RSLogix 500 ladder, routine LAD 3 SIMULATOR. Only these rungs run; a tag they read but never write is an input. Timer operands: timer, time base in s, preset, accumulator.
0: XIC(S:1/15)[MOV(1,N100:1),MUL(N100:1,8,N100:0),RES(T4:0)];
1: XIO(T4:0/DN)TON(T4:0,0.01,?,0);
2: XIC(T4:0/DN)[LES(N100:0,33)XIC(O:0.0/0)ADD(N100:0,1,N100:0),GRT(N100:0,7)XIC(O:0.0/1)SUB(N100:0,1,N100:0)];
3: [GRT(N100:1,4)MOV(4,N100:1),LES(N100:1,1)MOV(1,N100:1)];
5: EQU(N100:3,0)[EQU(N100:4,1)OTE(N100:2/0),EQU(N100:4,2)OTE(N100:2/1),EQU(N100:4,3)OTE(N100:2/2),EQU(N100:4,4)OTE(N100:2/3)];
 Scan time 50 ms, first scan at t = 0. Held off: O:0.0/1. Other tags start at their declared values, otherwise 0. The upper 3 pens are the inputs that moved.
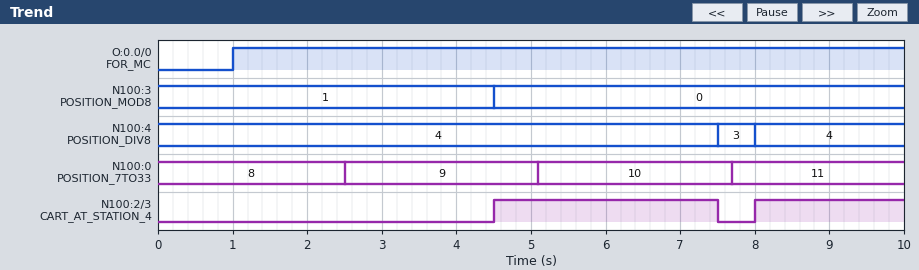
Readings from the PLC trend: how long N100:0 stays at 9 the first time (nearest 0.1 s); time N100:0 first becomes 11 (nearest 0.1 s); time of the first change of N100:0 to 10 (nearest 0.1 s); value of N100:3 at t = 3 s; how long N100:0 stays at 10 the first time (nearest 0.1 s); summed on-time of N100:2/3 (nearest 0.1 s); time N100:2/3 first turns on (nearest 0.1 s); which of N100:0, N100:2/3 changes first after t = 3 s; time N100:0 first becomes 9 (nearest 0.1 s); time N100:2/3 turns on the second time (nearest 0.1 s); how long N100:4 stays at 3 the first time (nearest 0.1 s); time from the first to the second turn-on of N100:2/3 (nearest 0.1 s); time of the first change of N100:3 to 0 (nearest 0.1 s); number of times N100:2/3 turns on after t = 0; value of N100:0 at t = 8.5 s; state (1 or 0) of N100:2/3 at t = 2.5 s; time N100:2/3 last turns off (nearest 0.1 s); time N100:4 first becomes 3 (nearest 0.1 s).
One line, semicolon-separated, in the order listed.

2.6 s; 7.7 s; 5.1 s; 1; 2.6 s; 5.0 s; 4.5 s; N100:2/3; 2.5 s; 8.0 s; 0.5 s; 3.5 s; 4.5 s; 2; 11; 0; 7.5 s; 7.5 s
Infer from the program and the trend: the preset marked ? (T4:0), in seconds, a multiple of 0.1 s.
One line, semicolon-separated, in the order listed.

2.5 s
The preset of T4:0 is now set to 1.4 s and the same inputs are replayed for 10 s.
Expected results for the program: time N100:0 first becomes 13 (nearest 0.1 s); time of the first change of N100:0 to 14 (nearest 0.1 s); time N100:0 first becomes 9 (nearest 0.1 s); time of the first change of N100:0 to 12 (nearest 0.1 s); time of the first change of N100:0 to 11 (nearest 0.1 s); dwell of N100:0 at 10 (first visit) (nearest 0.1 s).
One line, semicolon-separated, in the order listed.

7.4 s; 8.9 s; 1.4 s; 5.9 s; 4.4 s; 1.5 s
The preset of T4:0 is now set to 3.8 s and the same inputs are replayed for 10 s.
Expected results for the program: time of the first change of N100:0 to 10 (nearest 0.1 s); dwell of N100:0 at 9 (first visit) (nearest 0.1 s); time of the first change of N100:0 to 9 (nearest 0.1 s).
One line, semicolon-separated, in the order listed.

7.7 s; 3.9 s; 3.8 s
